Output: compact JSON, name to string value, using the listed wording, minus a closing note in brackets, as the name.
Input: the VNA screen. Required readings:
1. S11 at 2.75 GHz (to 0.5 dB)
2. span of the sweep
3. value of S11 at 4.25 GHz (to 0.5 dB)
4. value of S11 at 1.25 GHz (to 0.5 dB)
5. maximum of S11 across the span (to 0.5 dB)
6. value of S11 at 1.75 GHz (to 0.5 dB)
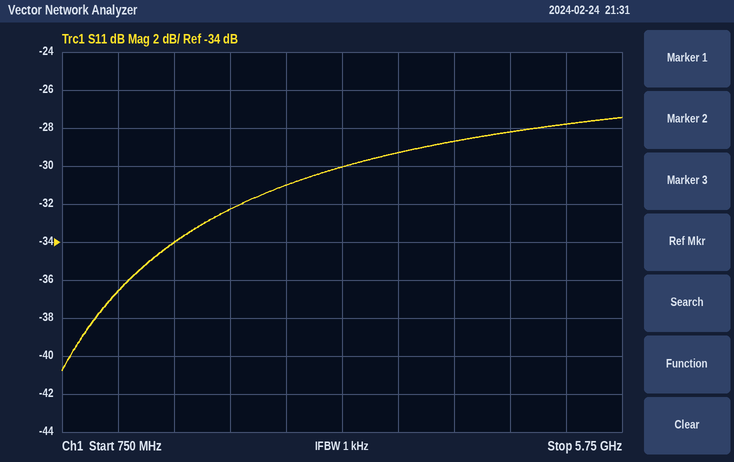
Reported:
{"S11 at 2.75 GHz": "-31.0 dB", "span of the sweep": "5 GHz", "value of S11 at 4.25 GHz": "-28.5 dB", "value of S11 at 1.25 GHz": "-36.5 dB", "maximum of S11 across the span": "-27.5 dB", "value of S11 at 1.75 GHz": "-34.0 dB"}
